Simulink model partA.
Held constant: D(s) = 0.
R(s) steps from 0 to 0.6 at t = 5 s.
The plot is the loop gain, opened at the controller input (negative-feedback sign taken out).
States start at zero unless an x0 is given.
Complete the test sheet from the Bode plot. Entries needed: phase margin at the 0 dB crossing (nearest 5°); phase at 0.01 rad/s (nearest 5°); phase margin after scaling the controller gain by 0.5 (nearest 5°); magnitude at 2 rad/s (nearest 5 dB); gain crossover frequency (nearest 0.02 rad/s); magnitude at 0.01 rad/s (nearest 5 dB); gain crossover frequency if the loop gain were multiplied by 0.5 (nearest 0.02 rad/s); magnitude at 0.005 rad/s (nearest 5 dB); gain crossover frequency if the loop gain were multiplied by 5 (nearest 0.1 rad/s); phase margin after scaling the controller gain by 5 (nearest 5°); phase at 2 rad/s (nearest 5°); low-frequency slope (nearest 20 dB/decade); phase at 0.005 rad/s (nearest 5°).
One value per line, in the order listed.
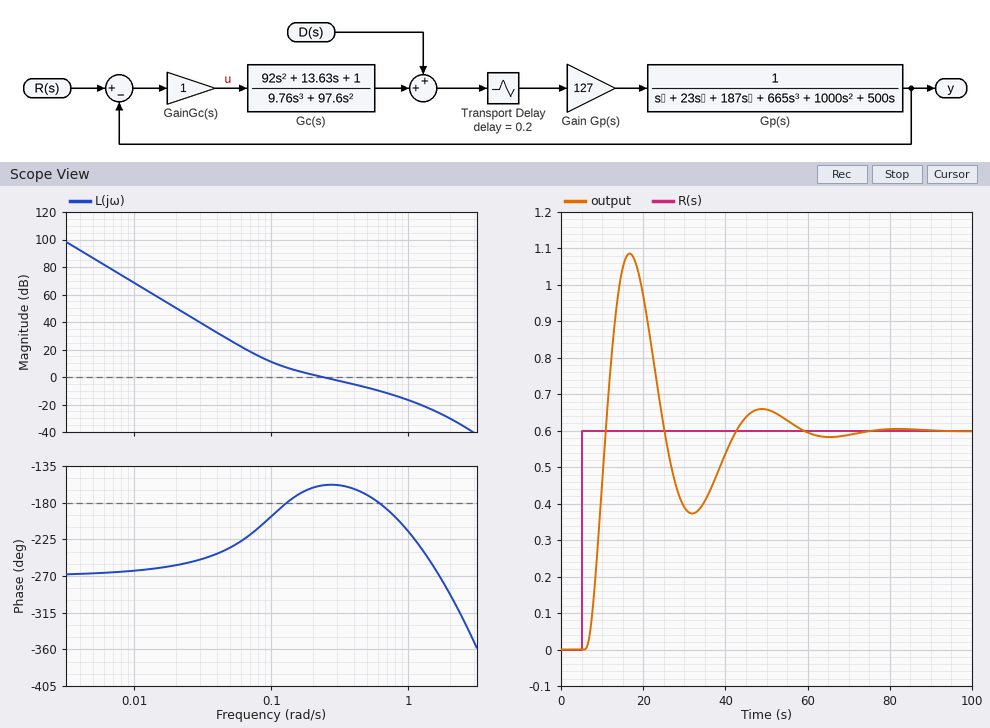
20°
-265°
5°
-30 dB
0.24 rad/s
70 dB
0.14 rad/s
85 dB
0.8 rad/s
-20°
-290°
-60 dB/decade
-265°
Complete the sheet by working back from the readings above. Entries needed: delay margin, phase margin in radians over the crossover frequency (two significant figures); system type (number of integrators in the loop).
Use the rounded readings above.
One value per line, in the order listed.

1.5 s
3
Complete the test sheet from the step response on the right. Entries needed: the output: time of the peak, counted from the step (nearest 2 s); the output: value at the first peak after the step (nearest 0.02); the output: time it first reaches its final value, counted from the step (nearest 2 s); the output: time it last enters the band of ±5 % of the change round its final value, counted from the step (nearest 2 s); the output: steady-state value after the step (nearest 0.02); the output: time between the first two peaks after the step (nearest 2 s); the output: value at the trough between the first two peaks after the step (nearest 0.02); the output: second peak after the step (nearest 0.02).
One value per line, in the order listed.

12 s
1.08
6 s
50 s
0.60
32 s
0.38
0.66
